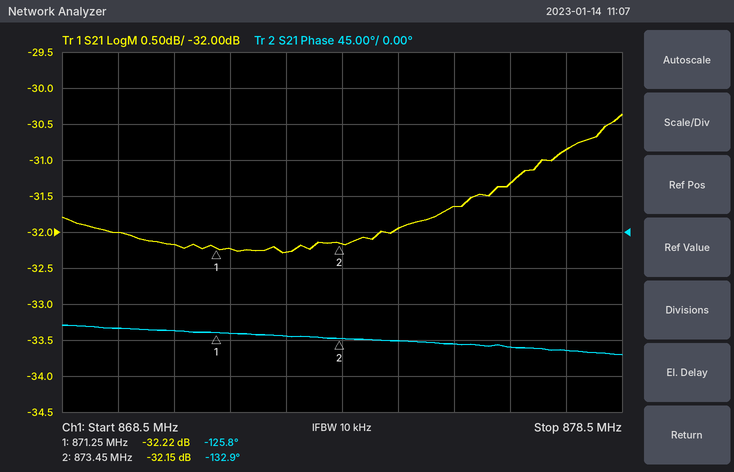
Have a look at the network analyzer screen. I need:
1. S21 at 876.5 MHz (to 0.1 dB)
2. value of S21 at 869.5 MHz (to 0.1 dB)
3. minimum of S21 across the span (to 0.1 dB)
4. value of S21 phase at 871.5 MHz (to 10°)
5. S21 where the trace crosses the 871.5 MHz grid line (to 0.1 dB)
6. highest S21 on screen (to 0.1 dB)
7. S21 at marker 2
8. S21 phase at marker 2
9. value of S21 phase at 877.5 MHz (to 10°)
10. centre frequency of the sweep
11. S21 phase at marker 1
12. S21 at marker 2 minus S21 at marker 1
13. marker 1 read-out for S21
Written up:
-31.3 dB
-32.0 dB
-32.3 dB
-130°
-32.2 dB
-30.4 dB
-32.15 dB
-132.9°
-150°
873.5 MHz
-125.8°
0.07 dB
-32.22 dB
